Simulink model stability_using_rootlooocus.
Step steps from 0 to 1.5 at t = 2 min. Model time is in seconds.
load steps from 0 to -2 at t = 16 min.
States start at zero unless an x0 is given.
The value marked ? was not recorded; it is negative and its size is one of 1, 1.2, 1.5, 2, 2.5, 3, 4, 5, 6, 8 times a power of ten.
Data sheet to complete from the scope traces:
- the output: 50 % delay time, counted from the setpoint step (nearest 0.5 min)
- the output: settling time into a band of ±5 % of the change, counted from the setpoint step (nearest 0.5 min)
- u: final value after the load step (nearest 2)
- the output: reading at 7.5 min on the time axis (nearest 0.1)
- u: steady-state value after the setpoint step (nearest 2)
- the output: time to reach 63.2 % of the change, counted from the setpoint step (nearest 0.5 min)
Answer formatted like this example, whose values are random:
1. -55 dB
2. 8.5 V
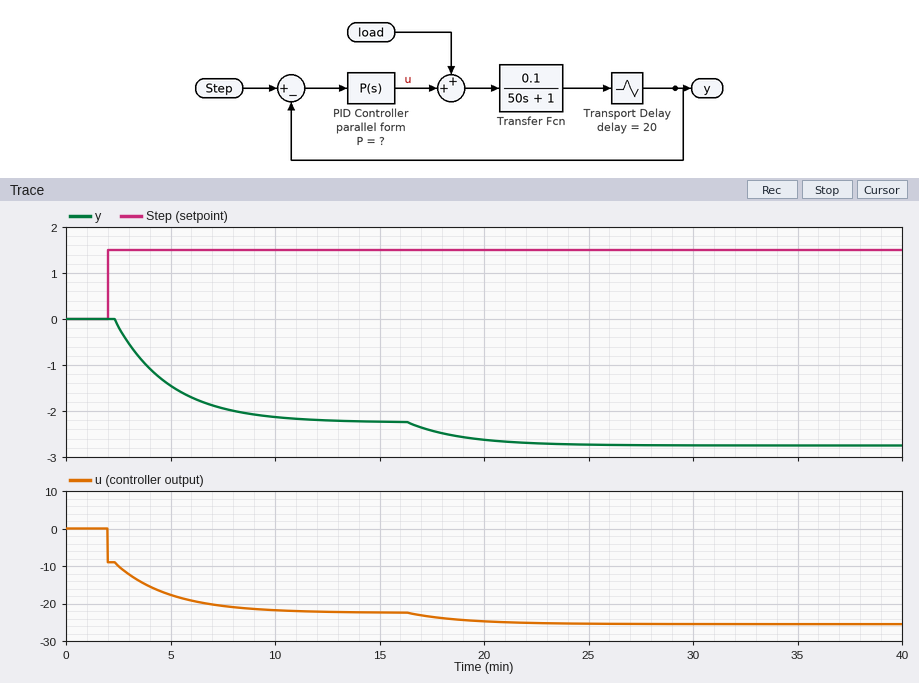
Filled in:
1. 2.0 min
2. 8.0 min
3. -26
4. -1.9
5. -22
6. 3.0 min
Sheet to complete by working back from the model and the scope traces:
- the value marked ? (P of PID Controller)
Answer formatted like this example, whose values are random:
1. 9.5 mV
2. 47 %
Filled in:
1. -6
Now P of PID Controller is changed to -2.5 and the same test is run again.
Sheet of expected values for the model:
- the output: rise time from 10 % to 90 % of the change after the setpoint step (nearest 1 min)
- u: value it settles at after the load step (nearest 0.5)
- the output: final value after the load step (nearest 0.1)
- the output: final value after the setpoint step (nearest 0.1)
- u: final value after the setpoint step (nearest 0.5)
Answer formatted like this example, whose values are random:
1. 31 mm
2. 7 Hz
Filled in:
1. 3 min
2. -5.5
3. -0.8
4. -0.5
5. -5.0
